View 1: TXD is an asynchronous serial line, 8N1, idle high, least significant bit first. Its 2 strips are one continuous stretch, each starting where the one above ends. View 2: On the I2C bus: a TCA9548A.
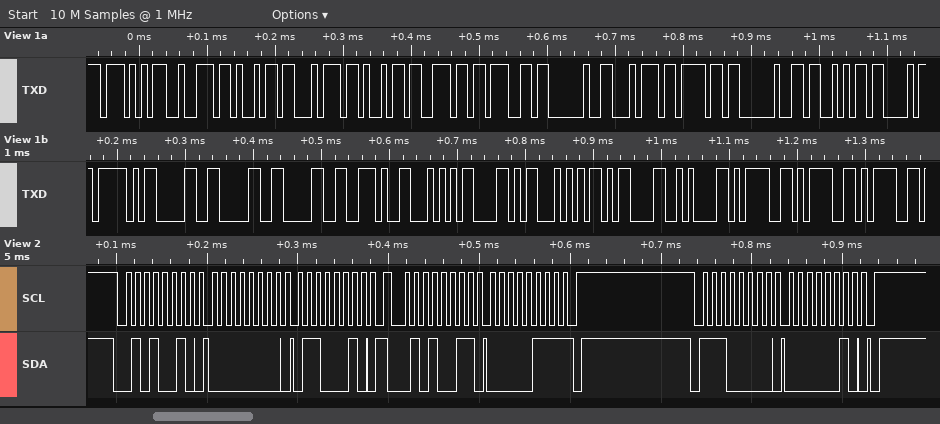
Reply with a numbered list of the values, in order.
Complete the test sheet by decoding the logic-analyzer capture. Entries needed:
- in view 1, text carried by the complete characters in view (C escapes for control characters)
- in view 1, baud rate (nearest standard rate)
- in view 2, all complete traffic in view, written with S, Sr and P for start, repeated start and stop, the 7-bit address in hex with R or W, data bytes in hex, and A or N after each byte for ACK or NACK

1. "Writing to SC_000.TXT\r\n==="
2. 115200 baud
3. S 29W A 00 A 62 A Sr 29R A 07 N P S 70W A 02 A P
